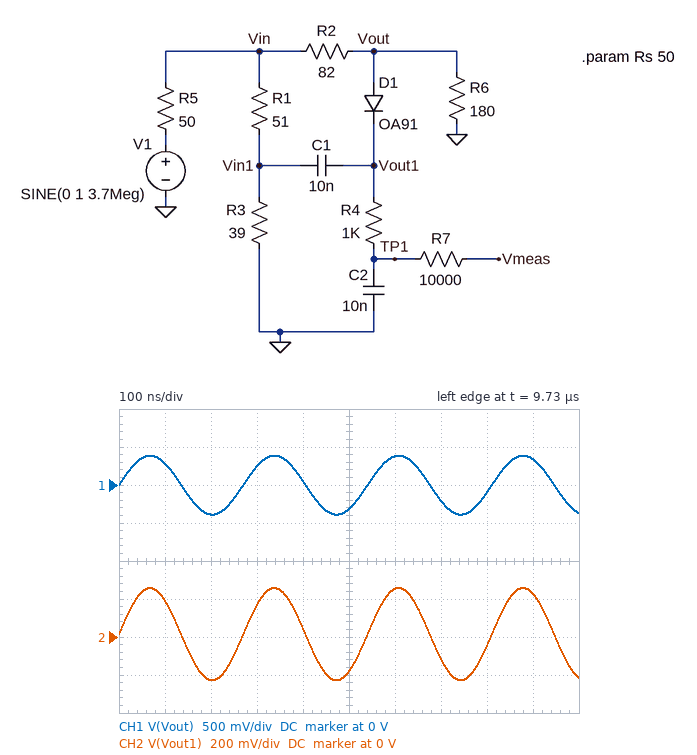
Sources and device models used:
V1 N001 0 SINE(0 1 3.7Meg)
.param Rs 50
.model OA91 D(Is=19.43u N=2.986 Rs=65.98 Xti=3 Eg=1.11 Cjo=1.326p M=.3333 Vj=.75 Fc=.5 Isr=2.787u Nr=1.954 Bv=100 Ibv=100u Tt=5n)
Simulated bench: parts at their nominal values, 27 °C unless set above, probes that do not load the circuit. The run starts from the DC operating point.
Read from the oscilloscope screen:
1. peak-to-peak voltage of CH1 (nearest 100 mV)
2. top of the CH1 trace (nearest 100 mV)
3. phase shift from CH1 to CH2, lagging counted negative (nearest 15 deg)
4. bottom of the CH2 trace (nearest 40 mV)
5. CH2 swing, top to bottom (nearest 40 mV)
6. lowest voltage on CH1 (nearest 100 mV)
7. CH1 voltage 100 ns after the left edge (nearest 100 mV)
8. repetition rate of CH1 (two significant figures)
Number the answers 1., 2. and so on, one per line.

1. 800 mV
2. 400 mV
3. 0 deg
4. -240 mV
5. 480 mV
6. -400 mV
7. 300 mV
8. 3.7 MHz
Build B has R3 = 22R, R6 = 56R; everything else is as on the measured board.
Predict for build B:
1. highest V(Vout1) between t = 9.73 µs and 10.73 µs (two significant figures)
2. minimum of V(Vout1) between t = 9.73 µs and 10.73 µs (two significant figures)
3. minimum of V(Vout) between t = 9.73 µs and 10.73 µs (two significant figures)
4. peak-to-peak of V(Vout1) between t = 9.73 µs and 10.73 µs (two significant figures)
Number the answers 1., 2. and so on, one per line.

1. 150 mV
2. -140 mV
3. -200 mV
4. 290 mV
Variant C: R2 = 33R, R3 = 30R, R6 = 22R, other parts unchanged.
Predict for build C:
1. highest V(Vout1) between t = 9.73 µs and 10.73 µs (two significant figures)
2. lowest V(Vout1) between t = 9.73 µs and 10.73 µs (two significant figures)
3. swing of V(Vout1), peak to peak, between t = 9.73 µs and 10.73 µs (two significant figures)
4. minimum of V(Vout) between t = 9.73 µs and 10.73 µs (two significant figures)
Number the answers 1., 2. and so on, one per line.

1. 140 mV
2. -140 mV
3. 290 mV
4. -160 mV
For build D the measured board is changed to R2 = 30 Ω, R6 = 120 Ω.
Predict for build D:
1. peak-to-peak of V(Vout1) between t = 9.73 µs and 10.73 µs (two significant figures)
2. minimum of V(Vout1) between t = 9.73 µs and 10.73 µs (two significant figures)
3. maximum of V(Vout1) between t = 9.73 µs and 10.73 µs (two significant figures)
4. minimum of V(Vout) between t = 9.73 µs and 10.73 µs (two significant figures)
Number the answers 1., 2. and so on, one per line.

1. 450 mV
2. -200 mV
3. 250 mV
4. -420 mV
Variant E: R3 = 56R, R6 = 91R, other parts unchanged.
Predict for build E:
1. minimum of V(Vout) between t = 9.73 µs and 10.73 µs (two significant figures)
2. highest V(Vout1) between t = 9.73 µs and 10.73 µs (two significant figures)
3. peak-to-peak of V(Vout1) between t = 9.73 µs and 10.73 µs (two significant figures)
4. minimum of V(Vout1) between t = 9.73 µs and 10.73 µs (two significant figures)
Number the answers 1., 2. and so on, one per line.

1. -300 mV
2. 290 mV
3. 580 mV
4. -290 mV
